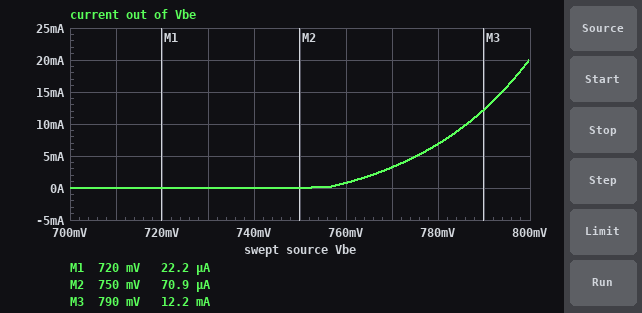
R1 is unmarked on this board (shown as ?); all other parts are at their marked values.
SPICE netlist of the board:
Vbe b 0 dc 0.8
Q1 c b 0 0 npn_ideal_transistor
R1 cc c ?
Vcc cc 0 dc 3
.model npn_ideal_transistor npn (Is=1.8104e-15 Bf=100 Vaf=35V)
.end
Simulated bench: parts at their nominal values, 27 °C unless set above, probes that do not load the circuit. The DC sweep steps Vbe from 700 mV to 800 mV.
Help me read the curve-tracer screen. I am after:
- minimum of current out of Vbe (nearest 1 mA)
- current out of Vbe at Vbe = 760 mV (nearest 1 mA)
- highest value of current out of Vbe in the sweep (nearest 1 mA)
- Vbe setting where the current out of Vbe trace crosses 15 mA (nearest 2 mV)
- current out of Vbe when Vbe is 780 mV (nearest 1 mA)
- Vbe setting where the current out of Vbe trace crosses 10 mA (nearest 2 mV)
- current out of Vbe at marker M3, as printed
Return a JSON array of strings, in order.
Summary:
["0 A", "1 mA", "20 mA", "794 mV", "7 mA", "786 mV", "12.2 mA"]
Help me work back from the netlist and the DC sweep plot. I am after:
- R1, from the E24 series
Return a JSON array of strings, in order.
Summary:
["330 Ω"]
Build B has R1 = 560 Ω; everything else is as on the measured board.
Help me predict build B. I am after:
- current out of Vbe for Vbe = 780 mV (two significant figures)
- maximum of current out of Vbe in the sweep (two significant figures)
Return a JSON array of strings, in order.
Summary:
["8.7 mA", "22 mA"]
